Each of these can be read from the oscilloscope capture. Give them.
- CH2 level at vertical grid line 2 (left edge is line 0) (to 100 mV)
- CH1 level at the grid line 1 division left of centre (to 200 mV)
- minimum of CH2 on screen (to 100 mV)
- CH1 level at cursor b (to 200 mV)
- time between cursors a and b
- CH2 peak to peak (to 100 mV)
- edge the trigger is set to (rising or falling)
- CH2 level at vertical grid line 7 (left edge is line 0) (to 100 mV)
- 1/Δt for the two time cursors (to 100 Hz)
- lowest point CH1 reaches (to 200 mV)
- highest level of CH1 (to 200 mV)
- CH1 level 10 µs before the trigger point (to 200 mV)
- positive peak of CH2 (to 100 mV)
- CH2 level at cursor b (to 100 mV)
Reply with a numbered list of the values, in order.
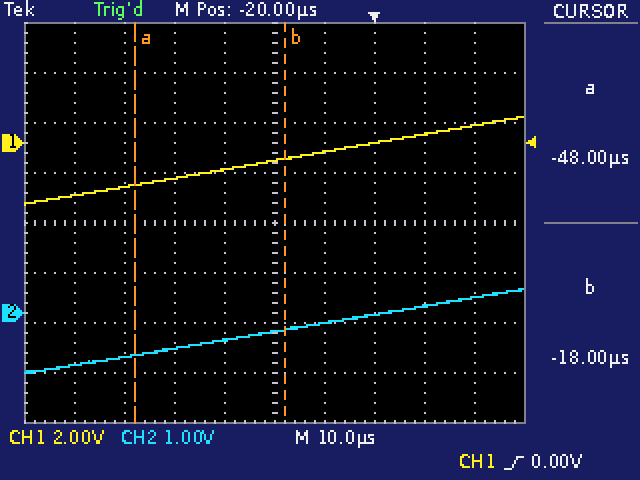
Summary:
1. -900 mV
2. -1.0 V
3. -1.2 V
4. -600 mV
5. 30 µs
6. 1.7 V
7. rising
8. 0.0 V
9. 33.3 kHz
10. -2.4 V
11. 1.0 V
12. -400 mV
13. 500 mV
14. -300 mV
